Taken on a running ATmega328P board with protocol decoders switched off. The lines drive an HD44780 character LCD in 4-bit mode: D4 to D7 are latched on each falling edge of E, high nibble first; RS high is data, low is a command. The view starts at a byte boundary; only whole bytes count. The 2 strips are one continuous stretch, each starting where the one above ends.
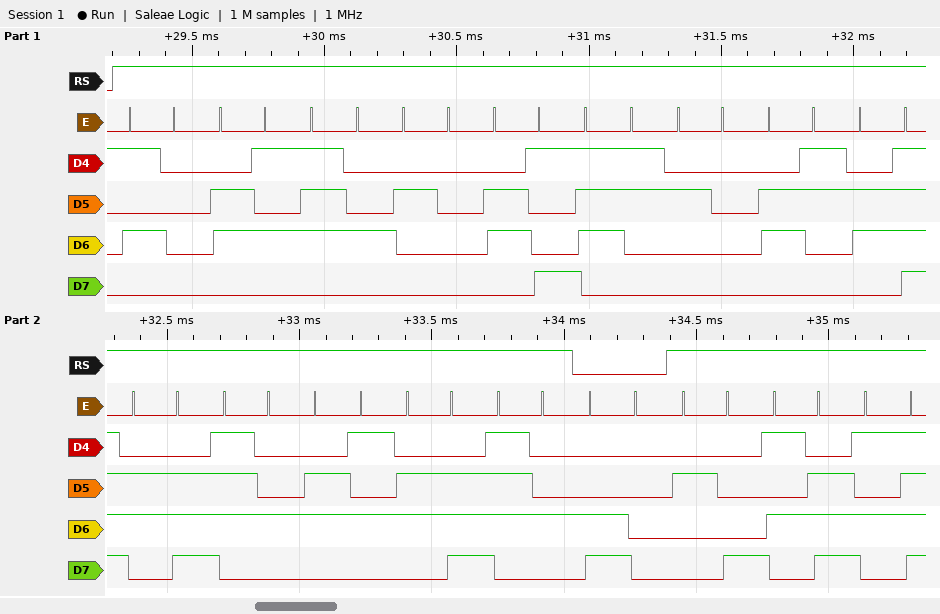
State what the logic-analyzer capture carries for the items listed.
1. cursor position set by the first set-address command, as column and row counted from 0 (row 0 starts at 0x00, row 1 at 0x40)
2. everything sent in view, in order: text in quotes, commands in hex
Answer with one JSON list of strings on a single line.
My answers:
["column 0, row 1", "\"Pet is content\" 0xC0 \"(^_\""]
